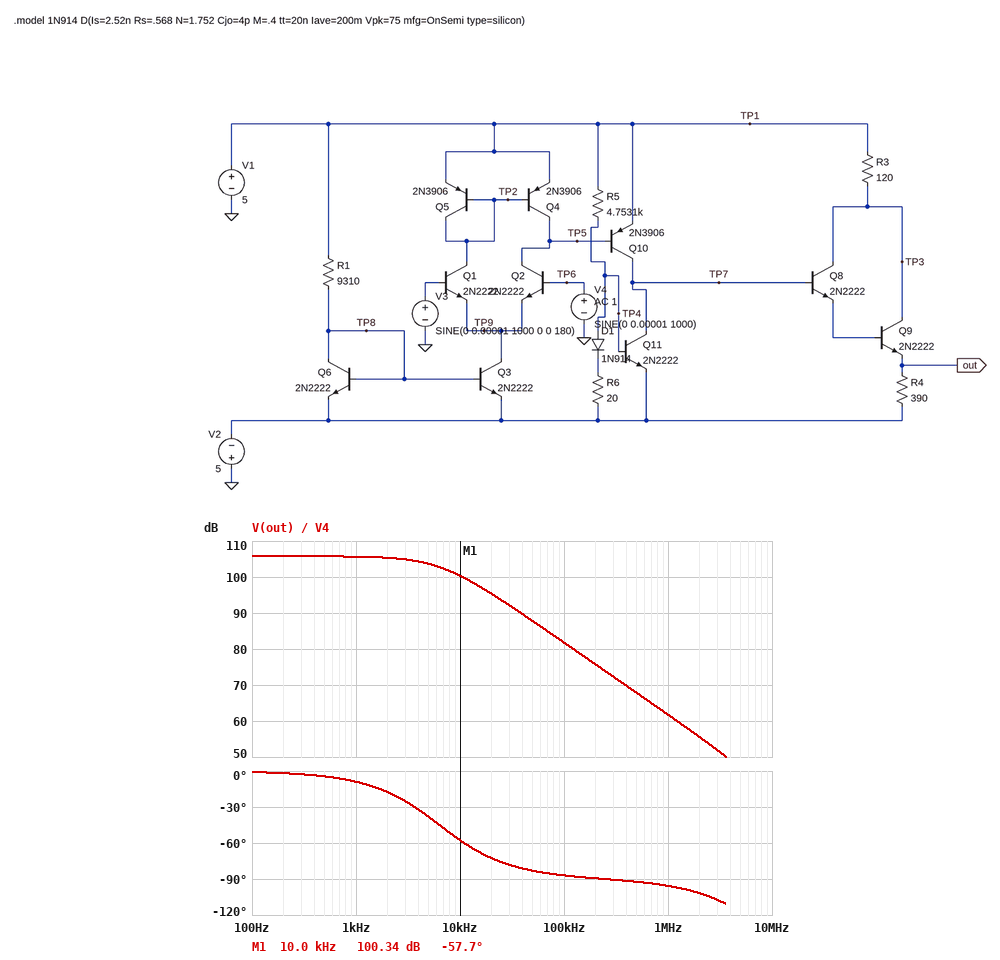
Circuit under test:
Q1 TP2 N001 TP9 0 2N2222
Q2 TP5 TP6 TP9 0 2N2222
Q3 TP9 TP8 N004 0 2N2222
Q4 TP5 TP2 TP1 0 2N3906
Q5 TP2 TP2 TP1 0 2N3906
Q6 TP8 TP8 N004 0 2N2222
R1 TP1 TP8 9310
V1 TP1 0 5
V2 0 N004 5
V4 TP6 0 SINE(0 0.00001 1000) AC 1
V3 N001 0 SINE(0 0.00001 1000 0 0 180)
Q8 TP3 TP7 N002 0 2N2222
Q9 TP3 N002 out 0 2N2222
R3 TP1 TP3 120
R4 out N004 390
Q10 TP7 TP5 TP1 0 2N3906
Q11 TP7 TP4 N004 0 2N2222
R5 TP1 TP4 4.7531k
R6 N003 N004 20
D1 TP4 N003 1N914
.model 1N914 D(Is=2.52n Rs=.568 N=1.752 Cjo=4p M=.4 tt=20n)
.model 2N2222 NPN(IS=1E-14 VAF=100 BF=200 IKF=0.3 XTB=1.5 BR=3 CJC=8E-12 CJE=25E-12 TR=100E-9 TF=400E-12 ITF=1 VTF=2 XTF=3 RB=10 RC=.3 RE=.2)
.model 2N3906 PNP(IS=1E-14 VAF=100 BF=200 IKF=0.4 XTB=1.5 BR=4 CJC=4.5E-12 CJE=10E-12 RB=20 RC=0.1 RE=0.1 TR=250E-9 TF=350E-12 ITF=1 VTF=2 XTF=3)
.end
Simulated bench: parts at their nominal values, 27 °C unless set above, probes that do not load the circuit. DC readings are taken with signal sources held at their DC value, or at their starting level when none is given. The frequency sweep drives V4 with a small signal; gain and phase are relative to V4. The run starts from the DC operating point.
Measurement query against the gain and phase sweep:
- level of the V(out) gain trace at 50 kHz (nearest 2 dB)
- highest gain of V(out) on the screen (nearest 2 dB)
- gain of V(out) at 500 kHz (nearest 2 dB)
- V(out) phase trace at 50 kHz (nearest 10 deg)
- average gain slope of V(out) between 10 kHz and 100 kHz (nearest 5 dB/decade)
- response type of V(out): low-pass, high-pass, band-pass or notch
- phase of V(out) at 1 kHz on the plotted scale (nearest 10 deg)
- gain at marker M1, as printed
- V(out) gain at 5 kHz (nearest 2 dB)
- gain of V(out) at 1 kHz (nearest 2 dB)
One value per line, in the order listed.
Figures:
88 dB
106 dB
68 dB
-80 deg
-20 dB/decade
low-pass
-10 deg
100.34 dB
104 dB
106 dB
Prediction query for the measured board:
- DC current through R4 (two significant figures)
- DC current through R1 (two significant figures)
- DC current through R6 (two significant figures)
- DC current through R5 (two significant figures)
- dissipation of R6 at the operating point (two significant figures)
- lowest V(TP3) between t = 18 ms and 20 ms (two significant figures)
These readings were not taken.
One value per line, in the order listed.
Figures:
9.0 mA
1.0 mA
2.0 mA
2.0 mA
77 µW
2.8 V
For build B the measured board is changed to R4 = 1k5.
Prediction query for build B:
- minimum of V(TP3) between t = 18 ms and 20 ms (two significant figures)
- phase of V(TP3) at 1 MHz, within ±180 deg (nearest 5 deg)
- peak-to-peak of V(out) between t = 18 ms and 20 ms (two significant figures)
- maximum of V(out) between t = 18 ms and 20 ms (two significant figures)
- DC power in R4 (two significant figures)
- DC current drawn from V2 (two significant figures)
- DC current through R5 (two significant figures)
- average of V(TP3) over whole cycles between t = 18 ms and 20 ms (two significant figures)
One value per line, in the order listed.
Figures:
4.4 V
80 deg
7.3 V
2.3 V
8.6 mW
7.4 mA
2.0 mA
4.7 V
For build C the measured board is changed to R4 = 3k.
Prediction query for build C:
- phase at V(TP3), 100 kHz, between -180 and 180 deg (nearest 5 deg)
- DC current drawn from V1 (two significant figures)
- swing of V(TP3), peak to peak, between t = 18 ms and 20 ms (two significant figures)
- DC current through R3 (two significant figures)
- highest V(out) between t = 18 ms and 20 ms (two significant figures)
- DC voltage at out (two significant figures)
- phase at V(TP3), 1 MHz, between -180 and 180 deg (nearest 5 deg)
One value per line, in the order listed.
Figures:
90 deg
6.2 mA
290 mV
1.2 mA
2.3 V
-1.4 V
75 deg
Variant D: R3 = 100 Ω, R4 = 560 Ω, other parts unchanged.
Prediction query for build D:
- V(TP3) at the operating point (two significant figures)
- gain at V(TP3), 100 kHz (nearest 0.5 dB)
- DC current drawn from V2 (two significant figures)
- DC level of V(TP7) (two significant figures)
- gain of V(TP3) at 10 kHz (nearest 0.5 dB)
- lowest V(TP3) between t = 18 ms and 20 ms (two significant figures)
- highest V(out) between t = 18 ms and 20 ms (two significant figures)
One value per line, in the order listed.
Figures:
4.4 V
67.0 dB
11 mA
-190 mV
85.5 dB
3.7 V
2.2 V
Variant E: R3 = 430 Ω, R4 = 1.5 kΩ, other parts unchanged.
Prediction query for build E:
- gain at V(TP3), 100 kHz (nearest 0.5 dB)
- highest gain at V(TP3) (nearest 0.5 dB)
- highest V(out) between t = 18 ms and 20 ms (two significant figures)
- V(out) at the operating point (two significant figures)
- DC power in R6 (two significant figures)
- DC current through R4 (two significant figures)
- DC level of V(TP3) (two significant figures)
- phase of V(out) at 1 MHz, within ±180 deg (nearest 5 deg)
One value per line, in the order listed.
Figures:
71.0 dB
95.0 dB
2.2 V
-1.4 V
77 µW
2.4 mA
4.0 V
-100 deg
